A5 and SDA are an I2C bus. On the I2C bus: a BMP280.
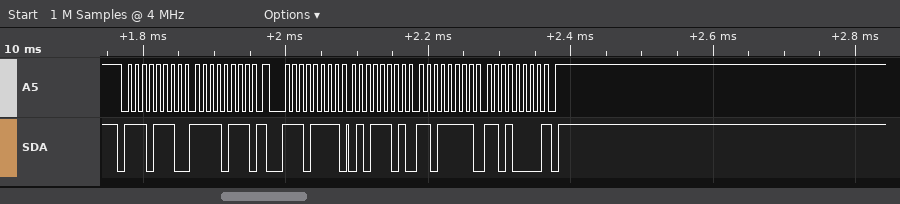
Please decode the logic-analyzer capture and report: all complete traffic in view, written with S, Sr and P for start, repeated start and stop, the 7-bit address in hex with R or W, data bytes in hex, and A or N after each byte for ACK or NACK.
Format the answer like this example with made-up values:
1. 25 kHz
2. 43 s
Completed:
1. S 77W A F7 A Sr 77R A 5D A DF A D0 N P
